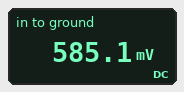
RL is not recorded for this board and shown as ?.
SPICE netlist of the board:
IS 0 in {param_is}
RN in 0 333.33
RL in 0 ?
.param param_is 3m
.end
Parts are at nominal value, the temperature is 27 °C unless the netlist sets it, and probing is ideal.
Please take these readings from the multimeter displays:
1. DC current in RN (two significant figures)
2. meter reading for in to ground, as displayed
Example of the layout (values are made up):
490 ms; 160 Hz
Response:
1.8 mA; 585.1 mV
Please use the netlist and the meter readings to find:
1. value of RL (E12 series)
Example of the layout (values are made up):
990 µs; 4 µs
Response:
470 Ω
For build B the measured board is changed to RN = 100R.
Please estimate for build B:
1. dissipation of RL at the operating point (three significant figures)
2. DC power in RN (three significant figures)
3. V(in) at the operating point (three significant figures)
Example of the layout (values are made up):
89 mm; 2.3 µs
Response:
130 µW; 612 µW; 247 mV
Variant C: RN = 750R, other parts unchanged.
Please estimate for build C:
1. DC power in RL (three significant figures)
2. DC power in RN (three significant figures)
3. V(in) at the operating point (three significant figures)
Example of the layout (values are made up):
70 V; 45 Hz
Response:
1.60 mW; 1.00 mW; 867 mV
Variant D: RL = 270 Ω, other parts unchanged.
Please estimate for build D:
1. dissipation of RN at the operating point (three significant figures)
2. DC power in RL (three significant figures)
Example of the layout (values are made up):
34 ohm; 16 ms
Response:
601 µW; 742 µW
